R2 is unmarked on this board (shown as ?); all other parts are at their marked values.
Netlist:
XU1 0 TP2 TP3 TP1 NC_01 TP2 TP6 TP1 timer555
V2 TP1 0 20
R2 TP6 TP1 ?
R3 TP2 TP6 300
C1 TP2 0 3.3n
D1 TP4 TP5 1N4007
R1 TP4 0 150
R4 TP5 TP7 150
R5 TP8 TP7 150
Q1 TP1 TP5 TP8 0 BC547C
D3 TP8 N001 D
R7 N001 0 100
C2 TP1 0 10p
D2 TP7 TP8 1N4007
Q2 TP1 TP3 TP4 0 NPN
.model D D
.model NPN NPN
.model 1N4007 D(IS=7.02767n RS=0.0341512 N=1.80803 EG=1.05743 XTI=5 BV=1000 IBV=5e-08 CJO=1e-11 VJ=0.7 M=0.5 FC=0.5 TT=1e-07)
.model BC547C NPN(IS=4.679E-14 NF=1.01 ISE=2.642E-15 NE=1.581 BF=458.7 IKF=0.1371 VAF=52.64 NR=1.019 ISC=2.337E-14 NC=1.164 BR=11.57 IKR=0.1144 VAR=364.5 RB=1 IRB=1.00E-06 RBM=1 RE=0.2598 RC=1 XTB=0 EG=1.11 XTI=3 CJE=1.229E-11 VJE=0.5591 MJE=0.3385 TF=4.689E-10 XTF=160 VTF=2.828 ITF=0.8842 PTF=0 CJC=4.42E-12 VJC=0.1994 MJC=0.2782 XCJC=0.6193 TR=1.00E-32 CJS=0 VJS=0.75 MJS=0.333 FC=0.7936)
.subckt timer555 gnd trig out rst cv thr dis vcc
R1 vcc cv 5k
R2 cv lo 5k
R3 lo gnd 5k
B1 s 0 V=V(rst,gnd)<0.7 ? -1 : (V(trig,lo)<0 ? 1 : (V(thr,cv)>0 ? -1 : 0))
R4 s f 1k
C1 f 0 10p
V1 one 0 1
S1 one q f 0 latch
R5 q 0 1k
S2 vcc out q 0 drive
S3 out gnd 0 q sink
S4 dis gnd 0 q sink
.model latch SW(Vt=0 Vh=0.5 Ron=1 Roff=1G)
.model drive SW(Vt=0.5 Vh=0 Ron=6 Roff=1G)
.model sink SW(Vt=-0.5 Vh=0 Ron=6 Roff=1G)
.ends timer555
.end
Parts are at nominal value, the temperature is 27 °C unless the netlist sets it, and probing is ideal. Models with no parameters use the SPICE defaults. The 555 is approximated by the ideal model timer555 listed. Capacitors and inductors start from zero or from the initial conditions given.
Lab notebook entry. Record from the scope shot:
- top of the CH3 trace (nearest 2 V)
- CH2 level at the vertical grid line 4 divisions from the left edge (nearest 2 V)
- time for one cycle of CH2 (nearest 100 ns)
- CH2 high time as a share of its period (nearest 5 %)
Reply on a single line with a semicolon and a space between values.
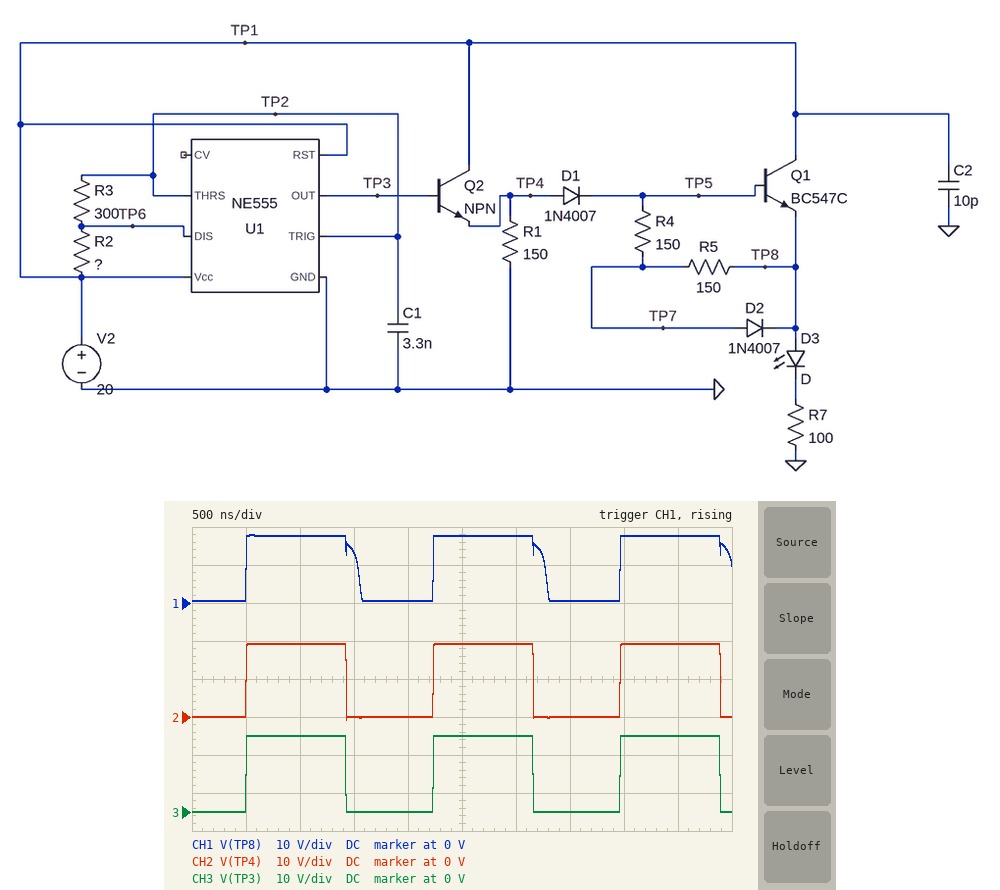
20 V; 0 V; 1.7 µs; 55 %
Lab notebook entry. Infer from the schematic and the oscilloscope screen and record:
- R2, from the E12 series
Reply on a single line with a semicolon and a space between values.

100 Ω
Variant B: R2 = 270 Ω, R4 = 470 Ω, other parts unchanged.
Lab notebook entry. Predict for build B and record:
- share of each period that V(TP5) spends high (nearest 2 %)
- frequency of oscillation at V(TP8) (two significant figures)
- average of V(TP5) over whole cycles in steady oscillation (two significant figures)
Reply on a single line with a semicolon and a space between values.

78 %; 490 kHz; 14 V
